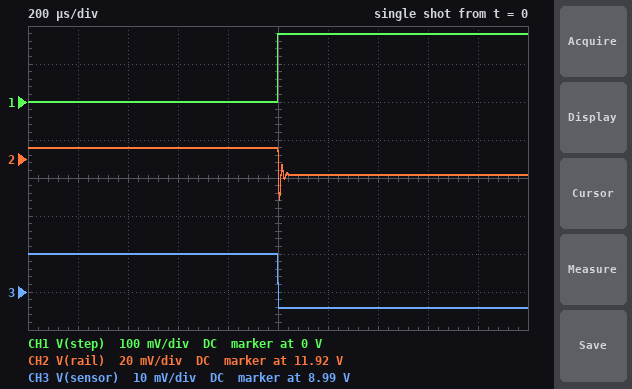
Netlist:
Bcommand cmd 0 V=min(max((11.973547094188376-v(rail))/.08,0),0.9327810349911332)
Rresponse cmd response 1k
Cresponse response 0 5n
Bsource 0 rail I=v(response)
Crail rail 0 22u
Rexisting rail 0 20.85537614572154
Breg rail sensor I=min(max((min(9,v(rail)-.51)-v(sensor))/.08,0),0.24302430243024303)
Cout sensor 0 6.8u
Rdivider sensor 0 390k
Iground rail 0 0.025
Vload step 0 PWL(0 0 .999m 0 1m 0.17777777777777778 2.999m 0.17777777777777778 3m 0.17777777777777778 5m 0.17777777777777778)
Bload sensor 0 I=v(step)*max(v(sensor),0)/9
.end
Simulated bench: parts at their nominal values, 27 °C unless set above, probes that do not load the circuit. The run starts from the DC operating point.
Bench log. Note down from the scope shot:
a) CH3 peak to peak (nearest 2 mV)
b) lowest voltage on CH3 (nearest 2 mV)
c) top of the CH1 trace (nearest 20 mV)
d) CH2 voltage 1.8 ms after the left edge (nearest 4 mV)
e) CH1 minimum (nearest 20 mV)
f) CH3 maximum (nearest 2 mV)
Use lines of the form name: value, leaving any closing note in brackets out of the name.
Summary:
CH3 peak to peak: 14 mV
lowest voltage on CH3: 8.986 V
top of the CH1 trace: 180 mV
CH2 voltage 1.8 ms after the left edge: 11.912 V
CH1 minimum: 0 V
CH3 maximum: 9.000 V
